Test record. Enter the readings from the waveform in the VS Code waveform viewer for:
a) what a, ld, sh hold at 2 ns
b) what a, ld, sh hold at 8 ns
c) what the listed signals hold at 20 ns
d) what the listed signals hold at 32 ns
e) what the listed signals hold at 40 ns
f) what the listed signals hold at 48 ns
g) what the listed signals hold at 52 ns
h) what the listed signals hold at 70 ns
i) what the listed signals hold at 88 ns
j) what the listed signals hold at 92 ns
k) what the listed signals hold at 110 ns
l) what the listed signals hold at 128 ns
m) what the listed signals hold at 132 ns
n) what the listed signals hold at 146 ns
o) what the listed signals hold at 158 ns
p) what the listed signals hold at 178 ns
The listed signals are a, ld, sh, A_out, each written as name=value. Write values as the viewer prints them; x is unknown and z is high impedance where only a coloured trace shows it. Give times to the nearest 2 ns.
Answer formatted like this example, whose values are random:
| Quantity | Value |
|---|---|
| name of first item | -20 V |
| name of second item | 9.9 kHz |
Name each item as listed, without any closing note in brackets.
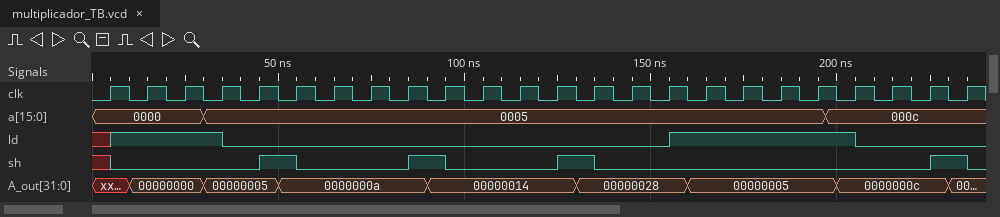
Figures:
| Quantity | Value |
|---|---|
| what a, ld, sh hold at 2 ns | a=0000, ld=x, sh=x |
| what a, ld, sh hold at 8 ns | a=0000, ld=1, sh=0 |
| what the listed signals hold at 20 ns | a=0000, ld=1, sh=0, A_out=00000000 |
| what the listed signals hold at 32 ns | a=0005, ld=1, sh=0, A_out=00000005 |
| what the listed signals hold at 40 ns | a=0005, ld=0, sh=0, A_out=00000005 |
| what the listed signals hold at 48 ns | a=0005, ld=0, sh=1, A_out=00000005 |
| what the listed signals hold at 52 ns | a=0005, ld=0, sh=1, A_out=0000000a |
| what the listed signals hold at 70 ns | a=0005, ld=0, sh=0, A_out=0000000a |
| what the listed signals hold at 88 ns | a=0005, ld=0, sh=1, A_out=0000000a |
| what the listed signals hold at 92 ns | a=0005, ld=0, sh=1, A_out=00000014 |
| what the listed signals hold at 110 ns | a=0005, ld=0, sh=0, A_out=00000014 |
| what the listed signals hold at 128 ns | a=0005, ld=0, sh=1, A_out=00000014 |
| what the listed signals hold at 132 ns | a=0005, ld=0, sh=1, A_out=00000028 |
| what the listed signals hold at 146 ns | a=0005, ld=0, sh=0, A_out=00000028 |
| what the listed signals hold at 158 ns | a=0005, ld=1, sh=0, A_out=00000028 |
| what the listed signals hold at 178 ns | a=0005, ld=1, sh=0, A_out=00000005 |
